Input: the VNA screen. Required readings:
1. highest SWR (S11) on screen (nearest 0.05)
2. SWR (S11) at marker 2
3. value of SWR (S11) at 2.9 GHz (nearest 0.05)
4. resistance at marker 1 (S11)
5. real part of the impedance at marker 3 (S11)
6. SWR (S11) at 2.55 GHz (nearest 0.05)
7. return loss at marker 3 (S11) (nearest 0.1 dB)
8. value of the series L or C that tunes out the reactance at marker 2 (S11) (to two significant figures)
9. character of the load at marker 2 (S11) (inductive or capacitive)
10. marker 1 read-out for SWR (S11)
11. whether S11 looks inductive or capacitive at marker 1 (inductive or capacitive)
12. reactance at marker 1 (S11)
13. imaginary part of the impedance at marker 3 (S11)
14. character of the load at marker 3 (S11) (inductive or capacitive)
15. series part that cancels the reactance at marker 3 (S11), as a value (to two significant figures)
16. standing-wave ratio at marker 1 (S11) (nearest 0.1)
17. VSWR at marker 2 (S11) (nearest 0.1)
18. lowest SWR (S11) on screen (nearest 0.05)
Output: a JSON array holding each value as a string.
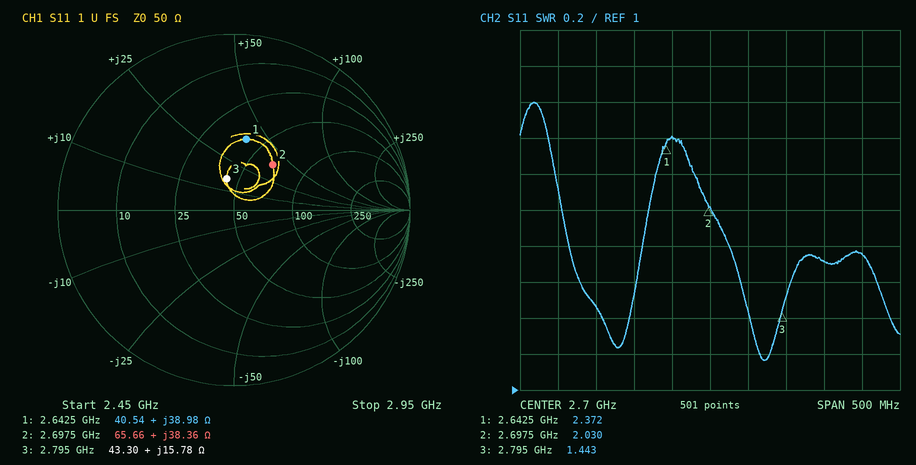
["2.60", "2.030", "1.75", "40.54 Ω", "43.30 Ω", "1.45", "14.8 dB", "1.5 pF", "inductive", "2.372", "inductive", "+38.98 Ω", "+15.78 Ω", "inductive", "3.6 pF", "2.4", "2.0", "1.15"]
